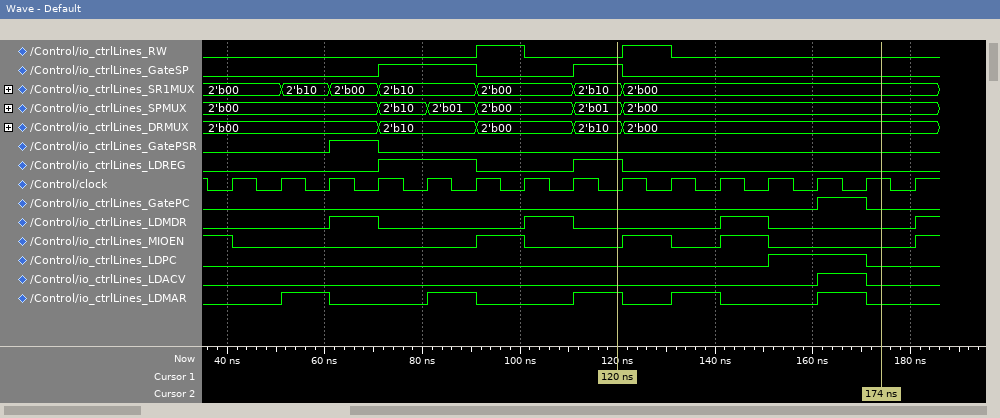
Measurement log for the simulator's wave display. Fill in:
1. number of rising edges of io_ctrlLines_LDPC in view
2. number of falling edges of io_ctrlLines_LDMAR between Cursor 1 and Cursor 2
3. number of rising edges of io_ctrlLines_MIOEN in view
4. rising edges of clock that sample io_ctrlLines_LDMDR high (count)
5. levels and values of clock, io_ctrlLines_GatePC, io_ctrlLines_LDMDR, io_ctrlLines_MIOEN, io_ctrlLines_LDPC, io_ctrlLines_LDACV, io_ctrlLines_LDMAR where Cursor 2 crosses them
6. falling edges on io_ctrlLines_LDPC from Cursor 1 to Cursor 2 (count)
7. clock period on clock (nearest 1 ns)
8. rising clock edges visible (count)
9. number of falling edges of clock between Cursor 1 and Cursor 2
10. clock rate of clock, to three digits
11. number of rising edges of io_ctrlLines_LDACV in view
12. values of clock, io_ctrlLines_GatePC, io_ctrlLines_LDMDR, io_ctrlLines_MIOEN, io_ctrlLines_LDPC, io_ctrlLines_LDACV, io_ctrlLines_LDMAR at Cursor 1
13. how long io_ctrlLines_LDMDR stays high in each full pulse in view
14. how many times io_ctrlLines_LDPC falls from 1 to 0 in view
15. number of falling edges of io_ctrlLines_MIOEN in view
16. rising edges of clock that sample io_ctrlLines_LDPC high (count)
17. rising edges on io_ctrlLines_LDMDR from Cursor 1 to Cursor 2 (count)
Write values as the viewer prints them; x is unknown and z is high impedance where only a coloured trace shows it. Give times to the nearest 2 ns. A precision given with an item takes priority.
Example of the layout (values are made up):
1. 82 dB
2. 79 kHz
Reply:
1. 1
2. 3
3. 4
4. 3
5. clock=1, io_ctrlLines_GatePC=0, io_ctrlLines_LDMDR=0, io_ctrlLines_MIOEN=0, io_ctrlLines_LDPC=0, io_ctrlLines_LDACV=0, io_ctrlLines_LDMAR=0
6. 1
7. 10 ns
8. 15
9. 5
10. 100 MHz
11. 1
12. clock=0, io_ctrlLines_GatePC=0, io_ctrlLines_LDMDR=0, io_ctrlLines_MIOEN=0, io_ctrlLines_LDPC=0, io_ctrlLines_LDACV=0, io_ctrlLines_LDMAR=1
13. 10 ns, 10 ns, 10 ns
14. 1
15. 4
16. 2
17. 1
